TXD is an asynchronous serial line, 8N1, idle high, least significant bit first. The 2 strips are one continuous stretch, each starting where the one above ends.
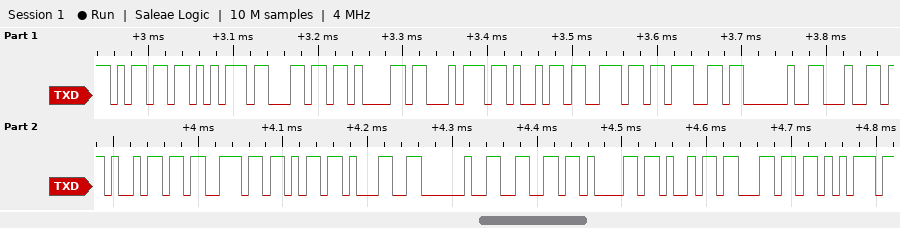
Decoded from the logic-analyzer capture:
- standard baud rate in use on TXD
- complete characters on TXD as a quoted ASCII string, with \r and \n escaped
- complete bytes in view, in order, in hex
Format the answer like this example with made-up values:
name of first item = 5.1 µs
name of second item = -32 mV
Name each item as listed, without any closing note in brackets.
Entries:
standard baud rate in use on TXD = 115200 baud
complete characters on TXD as a quoted ASCII string, with \r and \n escaped = "mulating disk1 failu"
complete bytes in view, in order, in hex = 6D 75 6C 61 74 69 6E 67 20 64 69 73 6B 31 20 66 61 69 6C 75
